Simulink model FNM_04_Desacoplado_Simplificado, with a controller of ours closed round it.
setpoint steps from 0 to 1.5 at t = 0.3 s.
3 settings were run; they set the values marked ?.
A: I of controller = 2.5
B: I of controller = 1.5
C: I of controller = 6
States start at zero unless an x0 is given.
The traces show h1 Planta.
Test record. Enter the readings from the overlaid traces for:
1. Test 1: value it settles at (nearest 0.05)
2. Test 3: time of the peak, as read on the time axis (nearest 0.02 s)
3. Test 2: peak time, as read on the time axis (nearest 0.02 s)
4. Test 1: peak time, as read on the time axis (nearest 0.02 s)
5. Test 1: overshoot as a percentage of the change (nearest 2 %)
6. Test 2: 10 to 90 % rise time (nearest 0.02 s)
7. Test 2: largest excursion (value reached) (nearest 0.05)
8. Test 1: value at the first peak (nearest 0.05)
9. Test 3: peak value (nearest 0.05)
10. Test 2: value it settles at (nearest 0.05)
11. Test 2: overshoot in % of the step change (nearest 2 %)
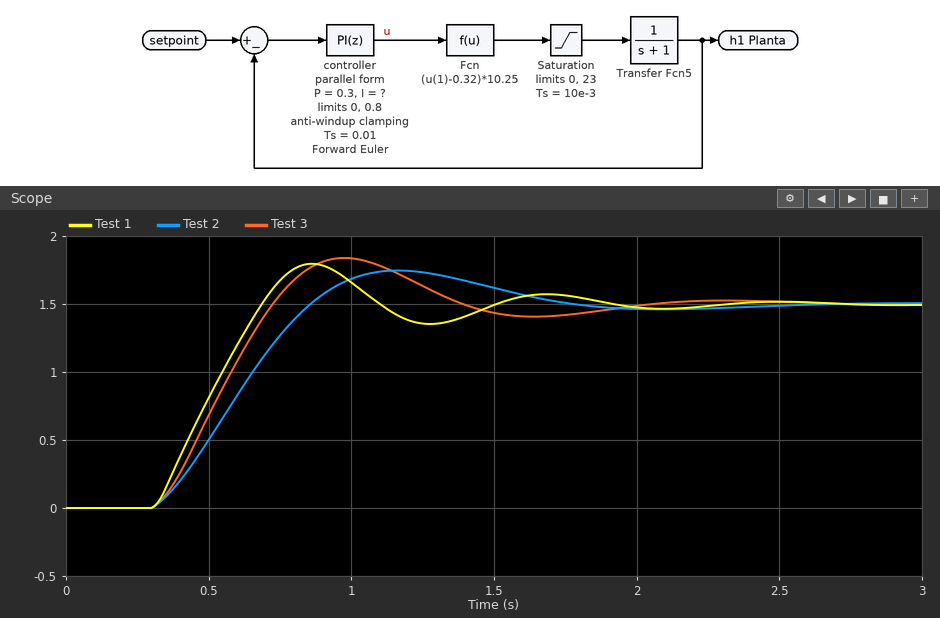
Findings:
1.50
0.98 s
1.16 s
0.86 s
20 %
0.40 s
1.75
1.80
1.85
1.50
16 %
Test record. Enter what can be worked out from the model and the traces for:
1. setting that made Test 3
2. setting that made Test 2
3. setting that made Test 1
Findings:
A
B
C
